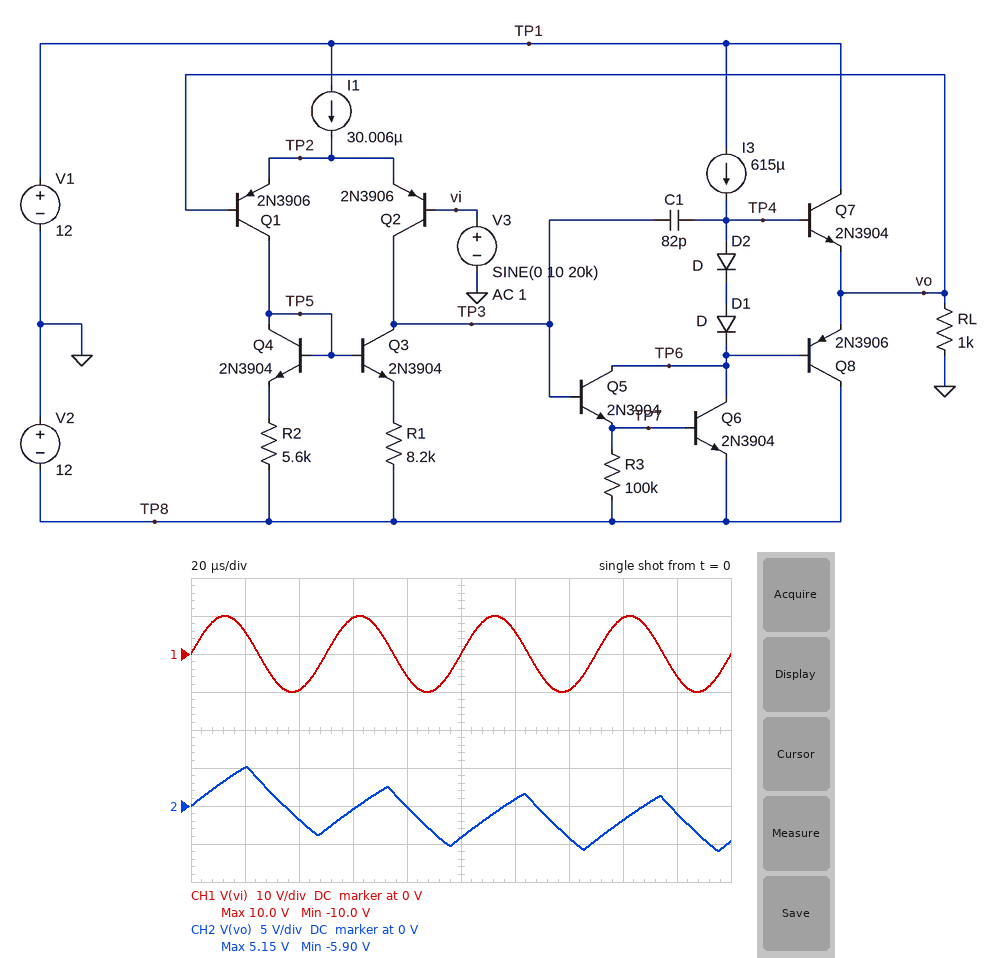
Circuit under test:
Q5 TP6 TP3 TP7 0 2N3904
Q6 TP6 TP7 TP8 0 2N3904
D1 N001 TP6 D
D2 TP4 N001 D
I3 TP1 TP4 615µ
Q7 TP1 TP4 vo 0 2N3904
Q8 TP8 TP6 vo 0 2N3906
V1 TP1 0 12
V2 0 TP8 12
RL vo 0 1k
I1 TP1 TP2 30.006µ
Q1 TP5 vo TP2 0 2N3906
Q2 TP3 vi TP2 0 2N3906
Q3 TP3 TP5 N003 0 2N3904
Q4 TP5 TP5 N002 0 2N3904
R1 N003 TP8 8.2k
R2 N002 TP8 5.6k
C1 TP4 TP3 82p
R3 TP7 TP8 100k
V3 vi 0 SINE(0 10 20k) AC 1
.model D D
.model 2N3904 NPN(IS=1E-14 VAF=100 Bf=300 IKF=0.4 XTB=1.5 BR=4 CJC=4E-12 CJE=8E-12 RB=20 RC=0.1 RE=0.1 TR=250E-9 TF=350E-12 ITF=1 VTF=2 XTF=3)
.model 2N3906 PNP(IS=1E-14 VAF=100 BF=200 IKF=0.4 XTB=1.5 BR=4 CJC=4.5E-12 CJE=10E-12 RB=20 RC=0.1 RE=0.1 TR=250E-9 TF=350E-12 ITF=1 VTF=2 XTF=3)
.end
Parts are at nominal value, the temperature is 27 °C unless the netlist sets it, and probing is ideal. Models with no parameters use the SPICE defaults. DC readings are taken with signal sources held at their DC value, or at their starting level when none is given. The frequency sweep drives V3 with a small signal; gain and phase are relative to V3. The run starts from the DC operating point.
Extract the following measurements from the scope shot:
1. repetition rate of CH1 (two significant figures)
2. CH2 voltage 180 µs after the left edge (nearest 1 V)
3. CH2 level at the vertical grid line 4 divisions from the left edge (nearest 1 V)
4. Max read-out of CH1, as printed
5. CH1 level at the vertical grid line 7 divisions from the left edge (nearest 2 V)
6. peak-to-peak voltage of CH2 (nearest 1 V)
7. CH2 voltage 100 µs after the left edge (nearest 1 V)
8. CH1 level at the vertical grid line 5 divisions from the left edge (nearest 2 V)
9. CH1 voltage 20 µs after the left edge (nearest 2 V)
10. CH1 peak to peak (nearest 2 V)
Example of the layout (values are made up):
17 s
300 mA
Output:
20 kHz
-1 V
0 V
10.0 V
-10 V
11 V
-4 V
0 V
6 V
20 V
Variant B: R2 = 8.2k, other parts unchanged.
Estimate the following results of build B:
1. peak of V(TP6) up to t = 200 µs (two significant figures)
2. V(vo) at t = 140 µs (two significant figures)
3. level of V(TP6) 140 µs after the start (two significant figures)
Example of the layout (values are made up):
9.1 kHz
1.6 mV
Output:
6.1 V
-2.3 V
-3.0 V
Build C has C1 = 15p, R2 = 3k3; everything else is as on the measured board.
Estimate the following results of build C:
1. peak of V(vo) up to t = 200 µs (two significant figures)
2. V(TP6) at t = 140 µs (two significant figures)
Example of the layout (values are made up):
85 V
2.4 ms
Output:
10 V
-10 V
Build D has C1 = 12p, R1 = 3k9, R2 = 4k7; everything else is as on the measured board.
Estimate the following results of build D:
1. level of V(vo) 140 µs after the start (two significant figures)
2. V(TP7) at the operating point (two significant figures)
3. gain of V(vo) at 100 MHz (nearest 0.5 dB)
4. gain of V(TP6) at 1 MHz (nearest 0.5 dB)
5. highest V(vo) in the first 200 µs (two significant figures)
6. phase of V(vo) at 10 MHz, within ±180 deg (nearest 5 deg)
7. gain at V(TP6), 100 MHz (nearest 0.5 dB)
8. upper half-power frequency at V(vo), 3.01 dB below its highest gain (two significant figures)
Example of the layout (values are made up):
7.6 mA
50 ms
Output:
-9.5 V
-11 V
-8.0 dB
0.5 dB
10 V
-150 deg
-10.0 dB
4.6 MHz
